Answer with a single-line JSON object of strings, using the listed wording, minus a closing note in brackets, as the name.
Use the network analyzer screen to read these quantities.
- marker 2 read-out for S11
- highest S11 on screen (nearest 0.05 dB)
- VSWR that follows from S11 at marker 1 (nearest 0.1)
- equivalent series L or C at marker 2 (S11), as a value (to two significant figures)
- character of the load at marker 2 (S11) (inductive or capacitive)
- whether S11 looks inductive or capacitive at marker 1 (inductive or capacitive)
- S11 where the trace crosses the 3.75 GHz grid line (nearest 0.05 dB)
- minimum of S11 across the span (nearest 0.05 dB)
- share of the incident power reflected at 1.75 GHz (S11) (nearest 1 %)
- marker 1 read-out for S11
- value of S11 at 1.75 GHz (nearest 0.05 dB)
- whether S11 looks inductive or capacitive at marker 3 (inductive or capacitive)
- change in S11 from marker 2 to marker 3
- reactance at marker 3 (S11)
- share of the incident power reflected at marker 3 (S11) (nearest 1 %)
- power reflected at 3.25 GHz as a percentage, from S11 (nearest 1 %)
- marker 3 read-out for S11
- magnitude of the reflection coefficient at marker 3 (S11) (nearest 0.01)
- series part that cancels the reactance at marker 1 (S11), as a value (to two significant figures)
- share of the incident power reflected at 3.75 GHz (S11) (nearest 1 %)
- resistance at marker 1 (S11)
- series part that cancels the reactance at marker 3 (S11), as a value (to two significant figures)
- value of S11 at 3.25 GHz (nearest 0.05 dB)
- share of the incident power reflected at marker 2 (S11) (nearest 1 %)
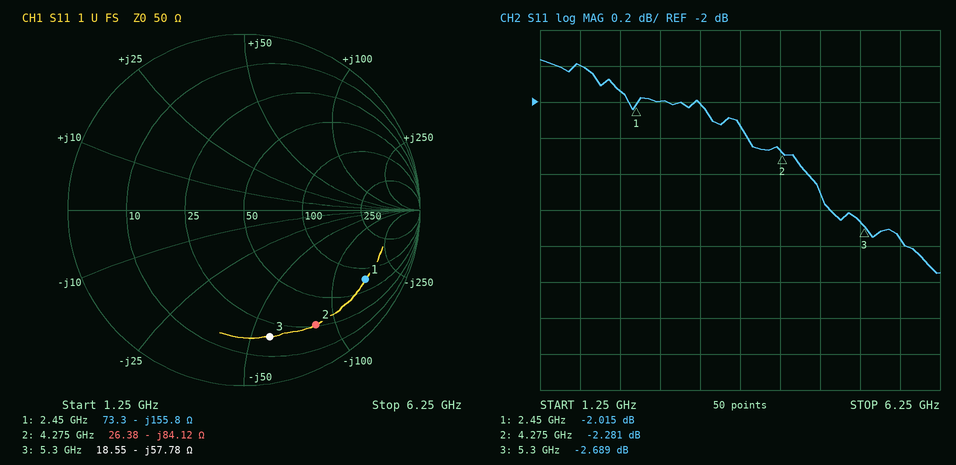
{"marker 2 read-out for S11": "-2.281 dB", "highest S11 on screen": "-1.75 dB", "VSWR that follows from S11 at marker 1": "8.7", "equivalent series L or C at marker 2 (S11), as a value": "440 fF", "character of the load at marker 2 (S11)": "capacitive", "whether S11 looks inductive or capacitive at marker 1": "capacitive", "S11 where the trace crosses the 3.75 GHz grid line": "-2.15 dB", "minimum of S11 across the span": "-2.95 dB", "share of the incident power reflected at 1.75 GHz (S11)": "66 %", "marker 1 read-out for S11": "-2.015 dB", "value of S11 at 1.75 GHz": "-1.80 dB", "whether S11 looks inductive or capacitive at marker 3": "capacitive", "change in S11 from marker 2 to marker 3": "-0.408 dB", "reactance at marker 3": "-57.78 Ω", "share of the incident power reflected at marker 3 (S11)": "54 %", "power reflected at 3.25 GHz as a percentage, from S11": "63 %", "marker 3 read-out for S11": "-2.689 dB", "magnitude of the reflection coefficient at marker 3 (S11)": "0.73", "series part that cancels the reactance at marker 1 (S11), as a value": "10 nH", "share of the incident power reflected at 3.75 GHz (S11)": "61 %", "resistance at marker 1": "73.3 Ω", "series part that cancels the reactance at marker 3 (S11), as a value": "1.7 nH", "value of S11 at 3.25 GHz": "-2.00 dB", "share of the incident power reflected at marker 2 (S11)": "59 %"}
